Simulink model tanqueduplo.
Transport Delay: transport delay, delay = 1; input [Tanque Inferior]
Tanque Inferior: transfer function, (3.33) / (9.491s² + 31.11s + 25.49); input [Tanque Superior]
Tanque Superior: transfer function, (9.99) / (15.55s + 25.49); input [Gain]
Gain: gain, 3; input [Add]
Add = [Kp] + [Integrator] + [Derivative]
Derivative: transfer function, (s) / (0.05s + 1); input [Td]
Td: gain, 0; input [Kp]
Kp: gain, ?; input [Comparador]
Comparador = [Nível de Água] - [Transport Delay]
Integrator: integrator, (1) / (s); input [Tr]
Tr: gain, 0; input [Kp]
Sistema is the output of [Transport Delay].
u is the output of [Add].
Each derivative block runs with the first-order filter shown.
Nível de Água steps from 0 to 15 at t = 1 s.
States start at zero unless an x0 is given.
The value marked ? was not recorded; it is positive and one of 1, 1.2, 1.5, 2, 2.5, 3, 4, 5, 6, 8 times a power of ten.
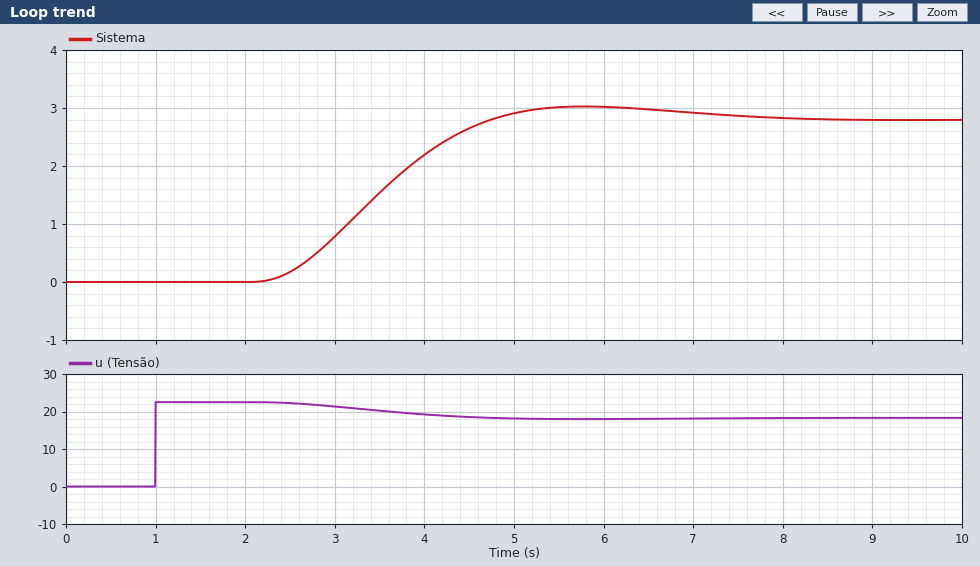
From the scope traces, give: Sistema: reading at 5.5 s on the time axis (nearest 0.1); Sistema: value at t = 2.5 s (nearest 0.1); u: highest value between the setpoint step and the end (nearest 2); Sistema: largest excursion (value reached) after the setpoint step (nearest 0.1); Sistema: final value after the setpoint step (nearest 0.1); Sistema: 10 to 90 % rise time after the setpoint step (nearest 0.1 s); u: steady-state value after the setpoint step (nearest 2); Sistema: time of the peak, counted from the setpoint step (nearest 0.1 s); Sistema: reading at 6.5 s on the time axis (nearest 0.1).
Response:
3.0
0.2
22
3.0
2.8
1.7 s
18
4.8 s
3.0
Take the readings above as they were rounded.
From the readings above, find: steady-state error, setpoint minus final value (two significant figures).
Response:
12
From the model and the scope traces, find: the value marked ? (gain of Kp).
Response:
1.5
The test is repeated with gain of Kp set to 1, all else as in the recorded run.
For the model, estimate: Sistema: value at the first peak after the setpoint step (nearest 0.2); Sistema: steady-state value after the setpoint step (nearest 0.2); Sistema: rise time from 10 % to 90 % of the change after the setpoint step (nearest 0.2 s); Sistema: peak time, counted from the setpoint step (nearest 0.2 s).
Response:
2.0
2.0
2.0 s
5.2 s
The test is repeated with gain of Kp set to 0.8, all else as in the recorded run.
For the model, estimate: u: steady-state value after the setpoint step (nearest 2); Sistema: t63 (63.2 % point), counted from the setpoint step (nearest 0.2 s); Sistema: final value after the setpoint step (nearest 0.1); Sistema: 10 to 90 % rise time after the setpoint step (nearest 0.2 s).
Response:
10
2.8 s
1.6
2.0 s
